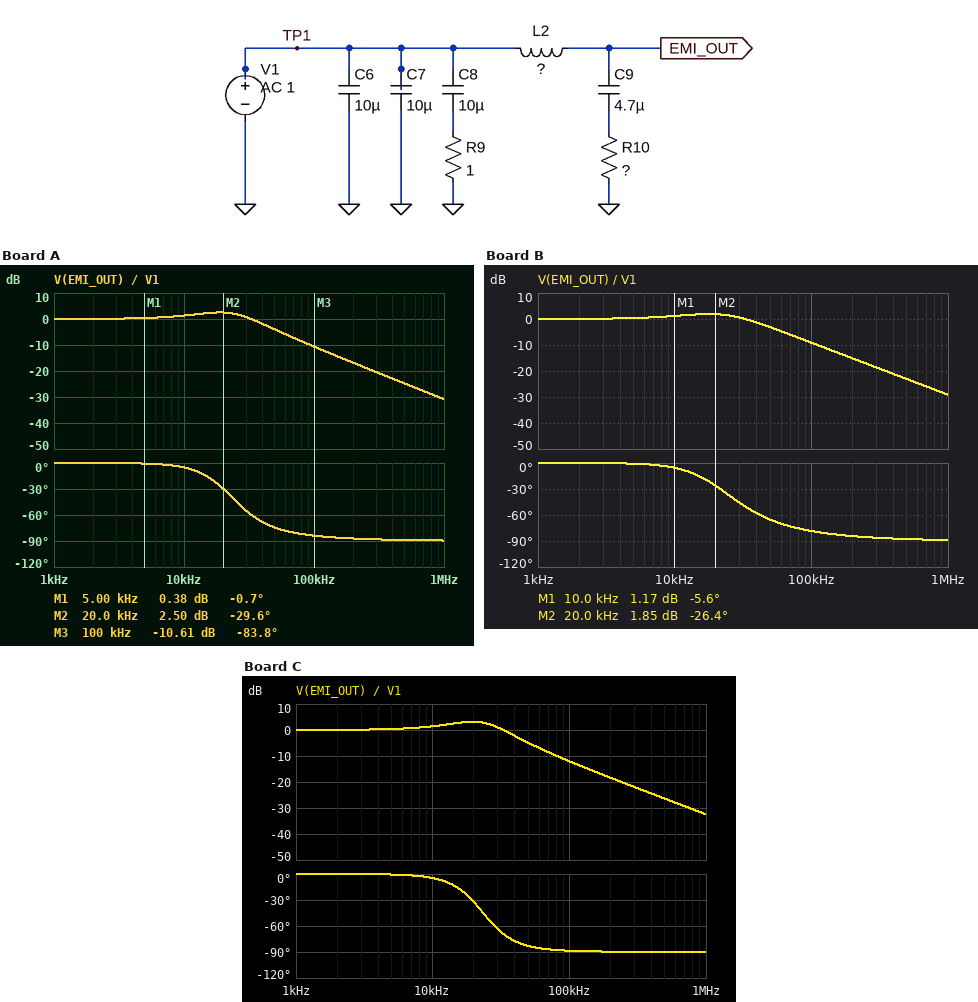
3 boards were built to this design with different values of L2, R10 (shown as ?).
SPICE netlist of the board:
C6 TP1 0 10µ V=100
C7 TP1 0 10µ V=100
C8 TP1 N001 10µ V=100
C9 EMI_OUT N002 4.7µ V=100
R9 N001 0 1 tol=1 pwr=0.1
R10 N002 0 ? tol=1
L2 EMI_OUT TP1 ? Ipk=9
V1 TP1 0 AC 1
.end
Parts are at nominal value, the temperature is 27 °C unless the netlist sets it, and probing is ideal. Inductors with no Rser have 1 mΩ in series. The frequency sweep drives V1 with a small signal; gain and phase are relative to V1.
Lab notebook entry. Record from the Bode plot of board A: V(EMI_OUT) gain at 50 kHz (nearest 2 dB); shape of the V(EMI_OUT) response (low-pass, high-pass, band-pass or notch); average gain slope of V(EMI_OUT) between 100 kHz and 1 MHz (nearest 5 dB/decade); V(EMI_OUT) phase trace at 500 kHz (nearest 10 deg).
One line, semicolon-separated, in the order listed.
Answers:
-4 dB; low-pass; -20 dB/decade; -90 deg
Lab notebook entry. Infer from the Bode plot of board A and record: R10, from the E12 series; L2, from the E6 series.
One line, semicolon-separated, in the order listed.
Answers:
1.8 Ω; 10 µH
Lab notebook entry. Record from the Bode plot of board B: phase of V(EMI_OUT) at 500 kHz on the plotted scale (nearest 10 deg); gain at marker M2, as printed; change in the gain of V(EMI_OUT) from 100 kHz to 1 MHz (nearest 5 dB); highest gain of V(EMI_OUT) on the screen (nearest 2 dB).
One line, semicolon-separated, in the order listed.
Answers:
-90 deg; 1.85 dB; -20 dB; 2 dB
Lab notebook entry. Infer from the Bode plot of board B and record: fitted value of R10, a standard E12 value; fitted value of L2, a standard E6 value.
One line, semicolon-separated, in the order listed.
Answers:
2.2 Ω; 10 µH
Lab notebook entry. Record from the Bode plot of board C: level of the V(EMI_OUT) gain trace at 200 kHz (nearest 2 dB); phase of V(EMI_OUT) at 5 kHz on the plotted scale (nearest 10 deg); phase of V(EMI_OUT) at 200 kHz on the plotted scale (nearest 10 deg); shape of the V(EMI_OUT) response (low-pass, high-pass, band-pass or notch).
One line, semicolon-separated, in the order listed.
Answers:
-18 dB; 0 deg; -90 deg; low-pass
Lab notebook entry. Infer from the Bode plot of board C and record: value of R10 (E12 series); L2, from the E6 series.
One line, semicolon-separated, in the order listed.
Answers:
1.5 Ω; 10 µH
